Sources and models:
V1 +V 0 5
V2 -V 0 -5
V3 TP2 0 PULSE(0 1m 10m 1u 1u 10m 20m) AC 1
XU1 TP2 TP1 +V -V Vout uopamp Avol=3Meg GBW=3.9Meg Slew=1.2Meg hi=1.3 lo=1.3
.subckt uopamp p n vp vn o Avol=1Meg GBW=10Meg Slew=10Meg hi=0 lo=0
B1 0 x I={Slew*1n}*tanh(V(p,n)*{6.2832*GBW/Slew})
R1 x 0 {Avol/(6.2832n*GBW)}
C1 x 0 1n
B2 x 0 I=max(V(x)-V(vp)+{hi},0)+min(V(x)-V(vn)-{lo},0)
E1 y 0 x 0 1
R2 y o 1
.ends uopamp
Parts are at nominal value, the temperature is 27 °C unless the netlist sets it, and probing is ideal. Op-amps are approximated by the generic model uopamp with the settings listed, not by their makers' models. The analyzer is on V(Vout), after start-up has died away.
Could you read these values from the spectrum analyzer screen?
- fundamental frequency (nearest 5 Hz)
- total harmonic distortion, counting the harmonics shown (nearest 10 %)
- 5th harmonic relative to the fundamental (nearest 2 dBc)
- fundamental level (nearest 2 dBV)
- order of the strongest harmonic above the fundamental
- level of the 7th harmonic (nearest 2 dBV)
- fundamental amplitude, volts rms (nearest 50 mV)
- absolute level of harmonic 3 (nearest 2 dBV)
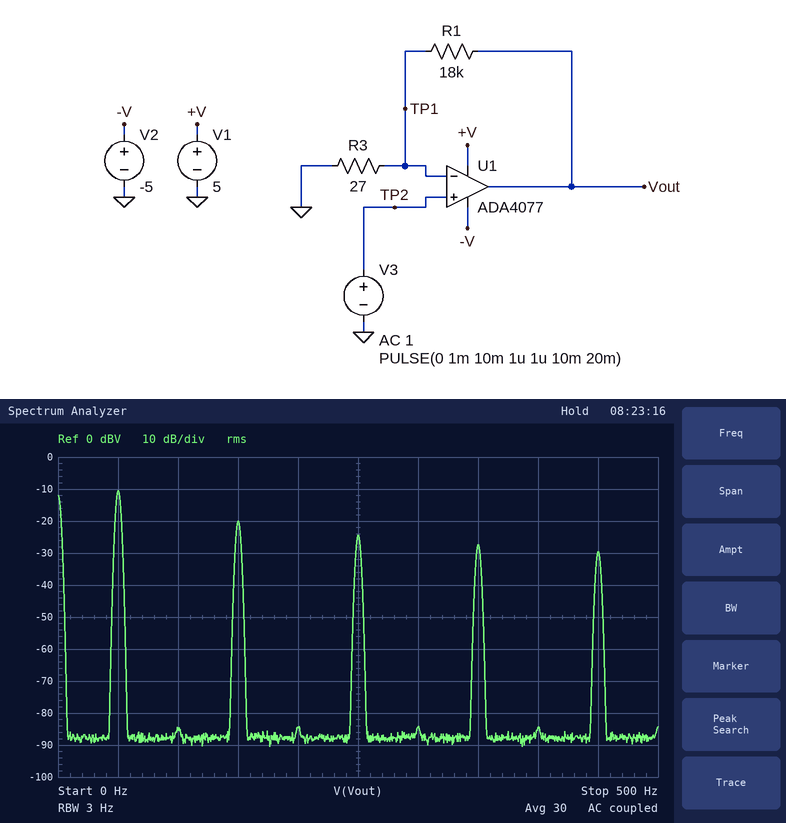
50 Hz
40 %
-14 dBc
-10 dBV
3
-28 dBV
300 mV
-20 dBV
